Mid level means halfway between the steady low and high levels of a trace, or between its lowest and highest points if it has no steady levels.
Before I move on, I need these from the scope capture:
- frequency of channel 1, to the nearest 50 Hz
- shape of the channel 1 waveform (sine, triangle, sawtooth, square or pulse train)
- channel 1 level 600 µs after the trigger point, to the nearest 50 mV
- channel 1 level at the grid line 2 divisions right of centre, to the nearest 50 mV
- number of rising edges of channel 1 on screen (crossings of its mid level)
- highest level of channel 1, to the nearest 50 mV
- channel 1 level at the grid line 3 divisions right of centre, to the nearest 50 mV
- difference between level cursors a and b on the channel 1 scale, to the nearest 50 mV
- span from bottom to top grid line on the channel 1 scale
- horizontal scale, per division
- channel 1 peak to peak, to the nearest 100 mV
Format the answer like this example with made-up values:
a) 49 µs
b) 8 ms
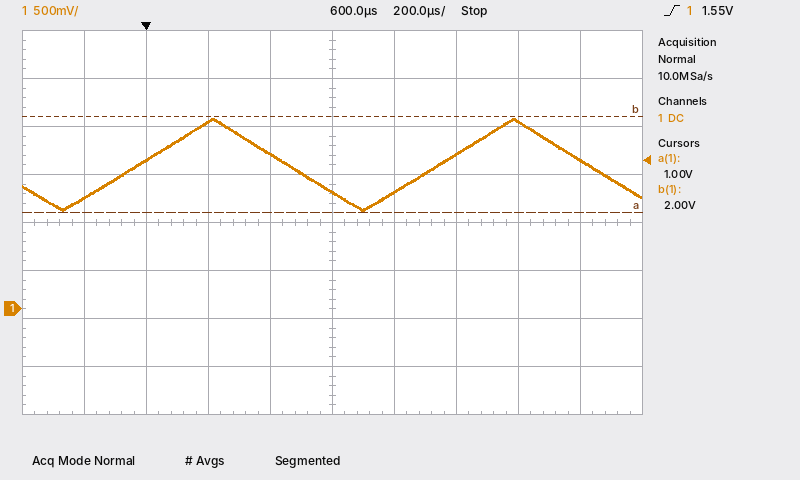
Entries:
a) 1.05 kHz
b) triangle
c) 1.20 V
d) 1.60 V
e) 2
f) 2.00 V
g) 1.95 V
h) 1.00 V
i) 4 V
j) 200 µs
k) 1.00 V
